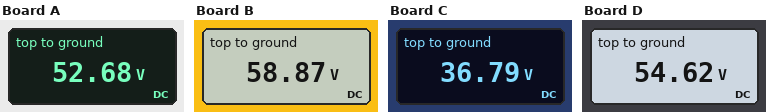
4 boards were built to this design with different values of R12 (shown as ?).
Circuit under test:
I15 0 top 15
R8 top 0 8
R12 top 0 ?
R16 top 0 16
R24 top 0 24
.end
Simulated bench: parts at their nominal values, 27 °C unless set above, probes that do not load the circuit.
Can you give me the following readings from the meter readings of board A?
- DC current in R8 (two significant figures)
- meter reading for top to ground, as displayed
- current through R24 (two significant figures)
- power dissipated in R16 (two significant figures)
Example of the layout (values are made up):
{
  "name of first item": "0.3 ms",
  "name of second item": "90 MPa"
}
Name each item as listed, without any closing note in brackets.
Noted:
{
  "DC current in R8": "6.6 A",
  "meter reading for top to ground, as displayed": "52.68 V",
  "current through R24": "2.2 A",
  "power dissipated in R16": "170 W"
}
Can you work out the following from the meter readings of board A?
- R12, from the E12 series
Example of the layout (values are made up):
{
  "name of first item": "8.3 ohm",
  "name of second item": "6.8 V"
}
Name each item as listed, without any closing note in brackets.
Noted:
{
  "R12, from the E12 series": "18 Ω"
}
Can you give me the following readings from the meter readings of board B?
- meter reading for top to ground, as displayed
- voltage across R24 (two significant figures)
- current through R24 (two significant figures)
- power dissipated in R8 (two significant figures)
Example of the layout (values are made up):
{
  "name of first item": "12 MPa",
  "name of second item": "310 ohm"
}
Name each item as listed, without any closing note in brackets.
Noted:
{
  "meter reading for top to ground, as displayed": "58.87 V",
  "voltage across R24": "59 V",
  "current through R24": "2.5 A",
  "power dissipated in R8": "430 W"
}
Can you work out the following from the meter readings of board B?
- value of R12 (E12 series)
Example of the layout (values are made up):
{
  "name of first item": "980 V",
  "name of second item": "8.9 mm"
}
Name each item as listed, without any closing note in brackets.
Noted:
{
  "value of R12": "39 Ω"
}
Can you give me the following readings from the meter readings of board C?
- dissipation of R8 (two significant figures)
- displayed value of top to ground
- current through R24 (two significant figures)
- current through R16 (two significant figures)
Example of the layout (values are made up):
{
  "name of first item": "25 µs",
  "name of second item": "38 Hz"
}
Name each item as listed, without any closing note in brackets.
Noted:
{
  "dissipation of R8": "170 W",
  "displayed value of top to ground": "36.79 V",
  "current through R24": "1.5 A",
  "current through R16": "2.3 A"
}
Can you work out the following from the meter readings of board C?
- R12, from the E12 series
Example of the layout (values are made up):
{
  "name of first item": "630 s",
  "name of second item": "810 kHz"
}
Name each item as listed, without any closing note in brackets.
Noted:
{
  "R12, from the E12 series": "5.6 Ω"
}
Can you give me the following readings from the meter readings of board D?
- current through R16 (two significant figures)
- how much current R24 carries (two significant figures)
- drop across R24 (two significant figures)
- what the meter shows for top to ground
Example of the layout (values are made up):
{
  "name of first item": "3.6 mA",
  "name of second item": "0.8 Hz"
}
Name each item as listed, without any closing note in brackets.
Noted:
{
  "current through R16": "3.4 A",
  "how much current R24 carries": "2.3 A",
  "drop across R24": "55 V",
  "what the meter shows for top to ground": "54.62 V"
}
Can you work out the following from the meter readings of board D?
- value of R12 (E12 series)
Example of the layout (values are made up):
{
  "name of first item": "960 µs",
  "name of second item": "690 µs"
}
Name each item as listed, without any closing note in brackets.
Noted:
{
  "value of R12": "22 Ω"
}
